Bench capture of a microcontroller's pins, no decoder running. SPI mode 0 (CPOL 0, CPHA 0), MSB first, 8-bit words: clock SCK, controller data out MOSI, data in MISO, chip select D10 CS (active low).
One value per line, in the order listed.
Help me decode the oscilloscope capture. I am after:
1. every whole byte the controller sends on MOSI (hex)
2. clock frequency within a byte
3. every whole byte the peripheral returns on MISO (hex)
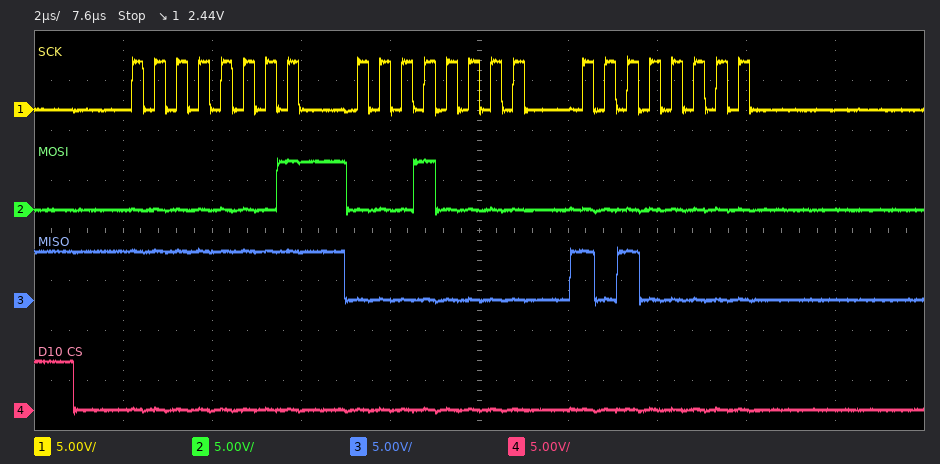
0x01 0x10 0x00
2 MHz
0xFF 0x00 0xA0
